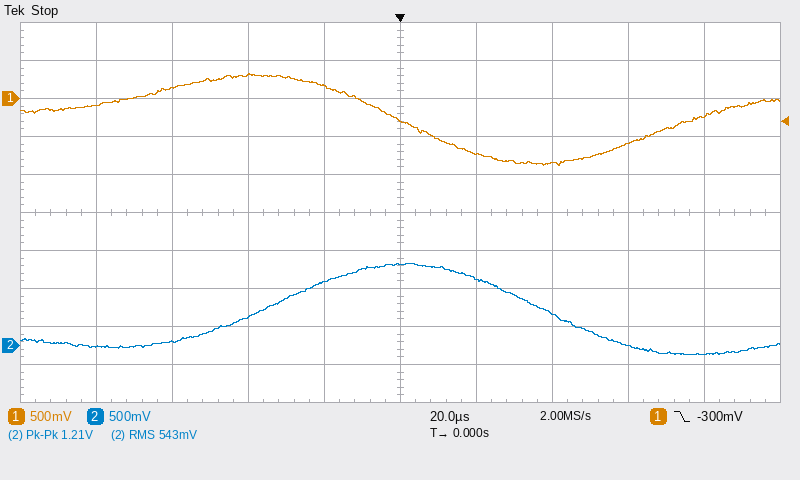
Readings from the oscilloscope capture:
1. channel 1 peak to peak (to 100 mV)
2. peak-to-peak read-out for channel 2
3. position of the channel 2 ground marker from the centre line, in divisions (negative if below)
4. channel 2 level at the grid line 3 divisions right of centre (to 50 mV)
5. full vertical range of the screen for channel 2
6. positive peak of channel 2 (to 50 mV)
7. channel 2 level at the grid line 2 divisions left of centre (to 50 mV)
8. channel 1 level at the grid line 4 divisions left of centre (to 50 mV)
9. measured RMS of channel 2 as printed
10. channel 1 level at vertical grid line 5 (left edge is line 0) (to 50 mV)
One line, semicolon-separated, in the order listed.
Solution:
1.20 V; 1.21 V; -3.5 div; 0 mV; 5 V; 1.10 V; 400 mV; -100 mV; 543 mV; -300 mV
